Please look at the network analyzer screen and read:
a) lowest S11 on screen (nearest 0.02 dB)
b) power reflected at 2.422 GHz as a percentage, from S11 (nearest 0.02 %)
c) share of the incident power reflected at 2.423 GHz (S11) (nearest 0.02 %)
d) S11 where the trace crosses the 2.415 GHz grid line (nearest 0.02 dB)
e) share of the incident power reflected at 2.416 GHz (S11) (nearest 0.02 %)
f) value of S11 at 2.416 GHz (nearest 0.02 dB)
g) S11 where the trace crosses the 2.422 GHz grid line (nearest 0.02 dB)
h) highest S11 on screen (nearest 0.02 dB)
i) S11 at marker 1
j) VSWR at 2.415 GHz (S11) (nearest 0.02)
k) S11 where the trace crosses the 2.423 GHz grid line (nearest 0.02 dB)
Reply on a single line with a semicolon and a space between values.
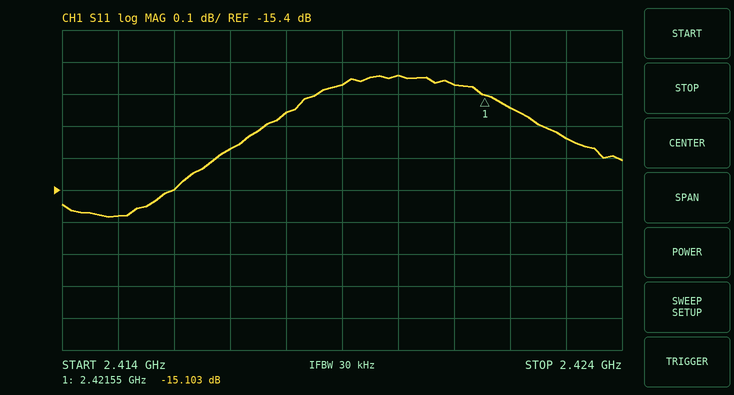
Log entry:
-15.48 dB; 3.06 %; 3.00 %; -15.48 dB; 2.88 %; -15.40 dB; -15.14 dB; -15.04 dB; -15.103 dB; 1.40; -15.24 dB
